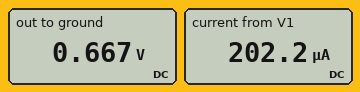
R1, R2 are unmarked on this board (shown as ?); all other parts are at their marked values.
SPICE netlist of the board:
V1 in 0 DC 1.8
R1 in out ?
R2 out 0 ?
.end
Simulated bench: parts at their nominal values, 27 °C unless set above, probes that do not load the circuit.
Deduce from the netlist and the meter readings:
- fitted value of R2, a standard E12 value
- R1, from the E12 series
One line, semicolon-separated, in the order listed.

3.3 kΩ; 5.6 kΩ
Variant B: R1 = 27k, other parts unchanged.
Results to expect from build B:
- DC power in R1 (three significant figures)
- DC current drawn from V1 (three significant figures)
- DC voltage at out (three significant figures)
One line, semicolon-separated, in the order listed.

95.3 µW; 59.4 µA; 196 mV
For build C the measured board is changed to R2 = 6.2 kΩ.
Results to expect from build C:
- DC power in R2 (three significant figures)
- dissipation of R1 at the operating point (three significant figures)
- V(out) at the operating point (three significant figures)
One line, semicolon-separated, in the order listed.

144 µW; 130 µW; 946 mV
